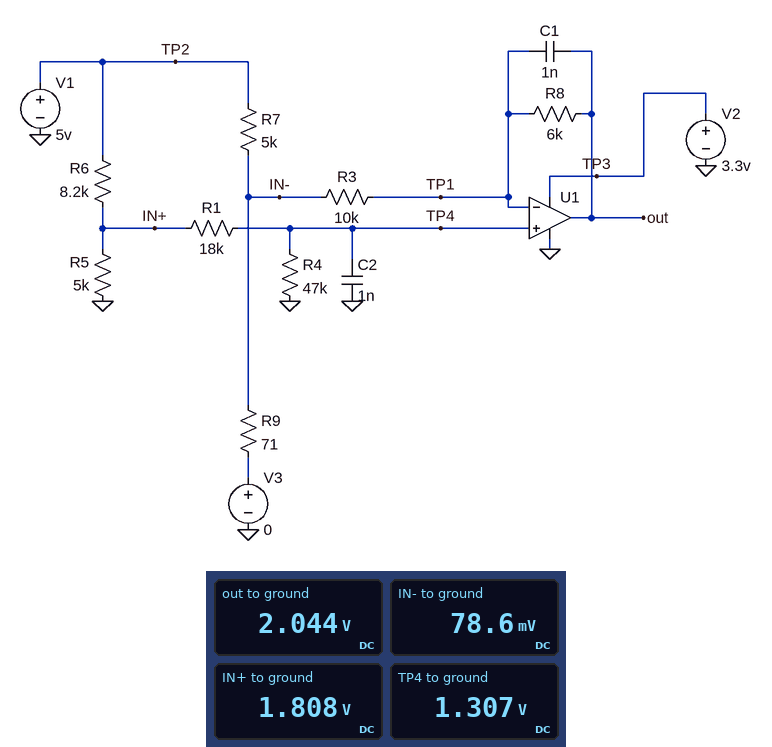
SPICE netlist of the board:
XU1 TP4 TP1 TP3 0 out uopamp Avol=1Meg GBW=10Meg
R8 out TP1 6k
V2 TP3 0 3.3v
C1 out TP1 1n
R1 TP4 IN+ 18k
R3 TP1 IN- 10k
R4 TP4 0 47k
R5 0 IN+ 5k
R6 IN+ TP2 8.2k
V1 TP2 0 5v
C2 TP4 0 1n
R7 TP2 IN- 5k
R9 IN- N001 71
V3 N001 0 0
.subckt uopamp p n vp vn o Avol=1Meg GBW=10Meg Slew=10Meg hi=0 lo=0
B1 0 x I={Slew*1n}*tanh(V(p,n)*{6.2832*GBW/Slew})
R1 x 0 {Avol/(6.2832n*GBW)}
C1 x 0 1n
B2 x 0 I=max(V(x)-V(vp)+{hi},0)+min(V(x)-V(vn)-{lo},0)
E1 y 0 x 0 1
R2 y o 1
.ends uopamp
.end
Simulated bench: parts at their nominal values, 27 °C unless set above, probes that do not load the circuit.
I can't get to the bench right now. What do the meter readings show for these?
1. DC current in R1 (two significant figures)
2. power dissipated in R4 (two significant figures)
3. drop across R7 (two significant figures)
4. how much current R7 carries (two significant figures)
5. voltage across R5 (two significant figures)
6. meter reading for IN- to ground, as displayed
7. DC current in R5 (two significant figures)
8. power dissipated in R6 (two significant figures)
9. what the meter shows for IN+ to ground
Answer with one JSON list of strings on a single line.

["28 µA", "36 µW", "4.9 V", "980 µA", "1.8 V", "78.6 mV", "360 µA", "1.2 mW", "1.808 V"]
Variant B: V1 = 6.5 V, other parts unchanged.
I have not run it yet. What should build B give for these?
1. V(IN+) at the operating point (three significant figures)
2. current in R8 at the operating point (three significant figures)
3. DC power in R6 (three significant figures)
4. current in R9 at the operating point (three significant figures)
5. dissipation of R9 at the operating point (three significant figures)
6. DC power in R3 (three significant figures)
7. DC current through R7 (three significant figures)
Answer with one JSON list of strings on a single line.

["2.35 V", "160 µA", "2.10 mW", "1.44 mA", "147 µW", "255 µW", "1.28 mA"]
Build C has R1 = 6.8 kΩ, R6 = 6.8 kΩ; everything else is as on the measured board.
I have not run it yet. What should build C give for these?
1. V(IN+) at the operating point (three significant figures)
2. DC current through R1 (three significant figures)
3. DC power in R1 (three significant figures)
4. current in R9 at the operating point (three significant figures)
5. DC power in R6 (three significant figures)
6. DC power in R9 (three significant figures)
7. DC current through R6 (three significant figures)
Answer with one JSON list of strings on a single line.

["2.01 V", "37.4 µA", "9.50 µW", "1.15 mA", "1.31 mW", "94.1 µW", "440 µA"]
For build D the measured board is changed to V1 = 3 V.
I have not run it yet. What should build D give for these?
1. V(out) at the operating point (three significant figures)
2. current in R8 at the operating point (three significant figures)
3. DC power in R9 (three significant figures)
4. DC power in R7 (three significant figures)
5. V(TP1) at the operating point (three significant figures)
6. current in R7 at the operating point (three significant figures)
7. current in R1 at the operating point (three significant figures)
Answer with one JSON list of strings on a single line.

["1.23 V", "73.7 µA", "31.3 µW", "1.74 mW", "784 mV", "591 µA", "16.7 µA"]
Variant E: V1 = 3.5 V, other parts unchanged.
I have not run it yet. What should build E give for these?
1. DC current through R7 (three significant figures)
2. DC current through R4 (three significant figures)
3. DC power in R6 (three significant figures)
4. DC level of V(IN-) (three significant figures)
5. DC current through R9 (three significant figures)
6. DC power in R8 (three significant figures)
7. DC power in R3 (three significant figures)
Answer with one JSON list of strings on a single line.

["689 µA", "19.5 µA", "609 µW", "55.0 mV", "775 µA", "44.4 µW", "73.9 µW"]
